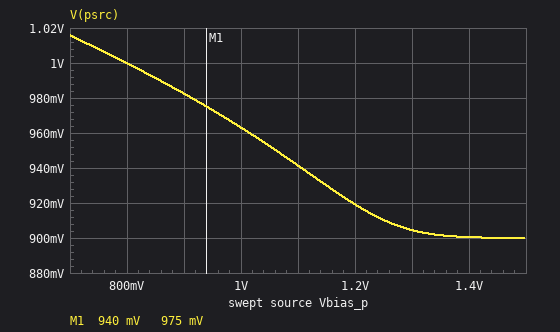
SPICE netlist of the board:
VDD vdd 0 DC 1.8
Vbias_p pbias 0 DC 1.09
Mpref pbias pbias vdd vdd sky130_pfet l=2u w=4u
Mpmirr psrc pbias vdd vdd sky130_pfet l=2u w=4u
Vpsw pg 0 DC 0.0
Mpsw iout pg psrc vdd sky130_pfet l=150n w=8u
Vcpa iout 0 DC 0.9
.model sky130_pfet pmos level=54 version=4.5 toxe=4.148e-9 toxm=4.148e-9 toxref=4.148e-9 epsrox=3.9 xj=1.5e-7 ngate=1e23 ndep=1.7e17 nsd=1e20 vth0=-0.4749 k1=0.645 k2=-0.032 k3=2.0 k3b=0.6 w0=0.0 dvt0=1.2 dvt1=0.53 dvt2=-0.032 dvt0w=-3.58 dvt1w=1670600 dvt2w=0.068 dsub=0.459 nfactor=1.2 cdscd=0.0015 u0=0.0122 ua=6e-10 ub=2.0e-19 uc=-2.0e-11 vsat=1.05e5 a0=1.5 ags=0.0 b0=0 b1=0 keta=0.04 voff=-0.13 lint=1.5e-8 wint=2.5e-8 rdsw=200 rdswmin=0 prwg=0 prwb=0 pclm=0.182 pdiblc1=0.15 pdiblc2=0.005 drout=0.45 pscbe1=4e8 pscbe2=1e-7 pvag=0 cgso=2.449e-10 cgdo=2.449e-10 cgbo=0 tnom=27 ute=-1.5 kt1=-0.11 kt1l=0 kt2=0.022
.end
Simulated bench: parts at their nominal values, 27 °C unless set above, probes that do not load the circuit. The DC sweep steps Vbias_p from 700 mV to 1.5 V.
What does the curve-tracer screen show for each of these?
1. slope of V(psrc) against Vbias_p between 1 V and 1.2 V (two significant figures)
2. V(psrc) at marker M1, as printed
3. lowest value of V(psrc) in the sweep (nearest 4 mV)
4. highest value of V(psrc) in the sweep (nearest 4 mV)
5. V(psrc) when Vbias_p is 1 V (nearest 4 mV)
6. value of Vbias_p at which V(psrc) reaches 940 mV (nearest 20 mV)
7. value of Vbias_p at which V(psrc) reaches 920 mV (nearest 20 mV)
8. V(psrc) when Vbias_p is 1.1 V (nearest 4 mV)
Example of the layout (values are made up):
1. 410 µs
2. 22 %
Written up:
1. -0.22 V/V
2. 975 mV
3. 900 mV
4. 1.016 V
5. 964 mV
6. 1.10 V
7. 1.20 V
8. 940 mV
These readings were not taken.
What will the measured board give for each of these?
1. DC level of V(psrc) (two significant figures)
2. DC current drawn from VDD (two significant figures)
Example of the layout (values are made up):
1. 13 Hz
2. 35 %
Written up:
1. 940 mV
2. 6.3 µA
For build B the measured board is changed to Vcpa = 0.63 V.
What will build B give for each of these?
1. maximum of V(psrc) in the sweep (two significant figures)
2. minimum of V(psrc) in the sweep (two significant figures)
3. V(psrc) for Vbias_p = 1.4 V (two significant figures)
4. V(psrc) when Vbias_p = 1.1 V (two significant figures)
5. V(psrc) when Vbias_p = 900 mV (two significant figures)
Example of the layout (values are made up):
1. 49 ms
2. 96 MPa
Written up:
1. 990 mV
2. 700 mV
3. 770 mV
4. 910 mV
5. 960 mV
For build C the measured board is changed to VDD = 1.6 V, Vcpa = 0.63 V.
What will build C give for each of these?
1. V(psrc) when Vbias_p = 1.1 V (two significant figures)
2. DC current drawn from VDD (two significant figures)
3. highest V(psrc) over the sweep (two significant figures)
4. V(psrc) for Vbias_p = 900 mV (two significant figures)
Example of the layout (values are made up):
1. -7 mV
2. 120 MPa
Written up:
1. 800 mV
2. 440 nA
3. 930 mV
4. 880 mV
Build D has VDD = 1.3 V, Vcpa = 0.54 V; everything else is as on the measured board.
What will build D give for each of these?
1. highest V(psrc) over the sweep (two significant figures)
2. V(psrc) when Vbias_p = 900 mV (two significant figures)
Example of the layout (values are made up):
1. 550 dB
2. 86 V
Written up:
1. 790 mV
2. 680 mV
